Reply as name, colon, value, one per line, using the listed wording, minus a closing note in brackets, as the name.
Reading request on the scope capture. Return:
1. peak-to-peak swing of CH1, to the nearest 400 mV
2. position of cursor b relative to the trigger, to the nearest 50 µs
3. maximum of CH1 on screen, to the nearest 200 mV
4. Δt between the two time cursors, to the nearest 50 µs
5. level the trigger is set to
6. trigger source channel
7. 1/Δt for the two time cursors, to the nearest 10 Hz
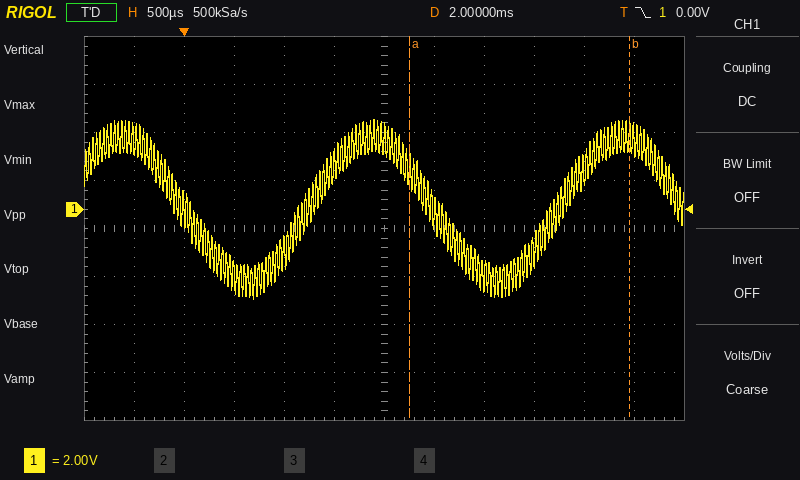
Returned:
peak-to-peak swing of CH1, to the nearest 400 mV: 7.6 V
position of cursor b relative to the trigger, to the nearest 50 µs: +4.45 ms
maximum of CH1 on screen, to the nearest 200 mV: 3.8 V
Δt between the two time cursors, to the nearest 50 µs: 2.20 ms
level the trigger is set to: 0.00 V
trigger source channel: CH1
1/Δt for the two time cursors, to the nearest 10 Hz: 450 Hz
